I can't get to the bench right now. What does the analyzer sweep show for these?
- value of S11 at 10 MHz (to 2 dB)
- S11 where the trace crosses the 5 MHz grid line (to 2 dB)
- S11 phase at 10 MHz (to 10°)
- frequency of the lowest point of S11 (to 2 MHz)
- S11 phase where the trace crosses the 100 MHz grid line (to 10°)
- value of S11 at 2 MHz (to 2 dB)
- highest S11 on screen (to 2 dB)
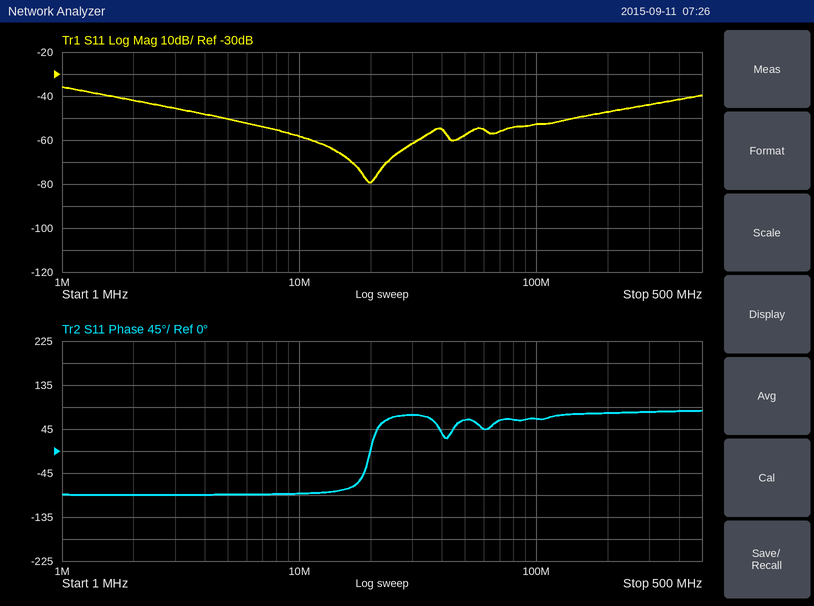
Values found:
-58 dB
-50 dB
-90°
20 MHz
70°
-42 dB
-36 dB
